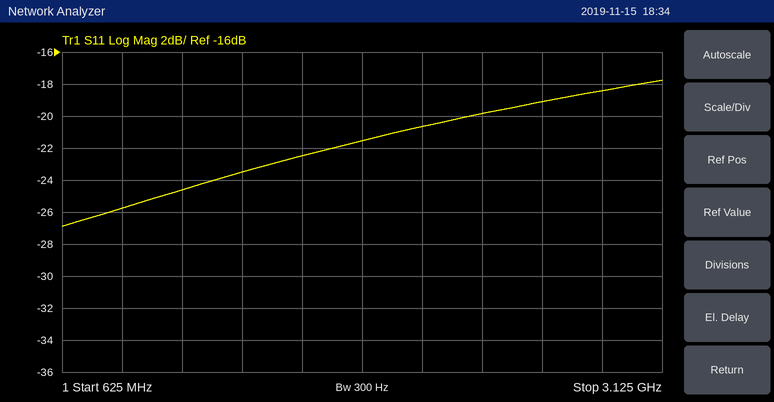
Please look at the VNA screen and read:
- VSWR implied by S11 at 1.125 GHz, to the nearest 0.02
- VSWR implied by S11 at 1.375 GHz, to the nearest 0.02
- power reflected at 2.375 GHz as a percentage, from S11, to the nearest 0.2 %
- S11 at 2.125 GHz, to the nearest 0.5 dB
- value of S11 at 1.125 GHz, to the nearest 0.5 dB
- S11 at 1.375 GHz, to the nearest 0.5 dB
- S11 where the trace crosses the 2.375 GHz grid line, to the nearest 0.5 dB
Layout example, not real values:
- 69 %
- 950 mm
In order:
- 1.12
- 1.14
- 1.0 %
- -20.5 dB
- -24.5 dB
- -23.5 dB
- -20.0 dB
